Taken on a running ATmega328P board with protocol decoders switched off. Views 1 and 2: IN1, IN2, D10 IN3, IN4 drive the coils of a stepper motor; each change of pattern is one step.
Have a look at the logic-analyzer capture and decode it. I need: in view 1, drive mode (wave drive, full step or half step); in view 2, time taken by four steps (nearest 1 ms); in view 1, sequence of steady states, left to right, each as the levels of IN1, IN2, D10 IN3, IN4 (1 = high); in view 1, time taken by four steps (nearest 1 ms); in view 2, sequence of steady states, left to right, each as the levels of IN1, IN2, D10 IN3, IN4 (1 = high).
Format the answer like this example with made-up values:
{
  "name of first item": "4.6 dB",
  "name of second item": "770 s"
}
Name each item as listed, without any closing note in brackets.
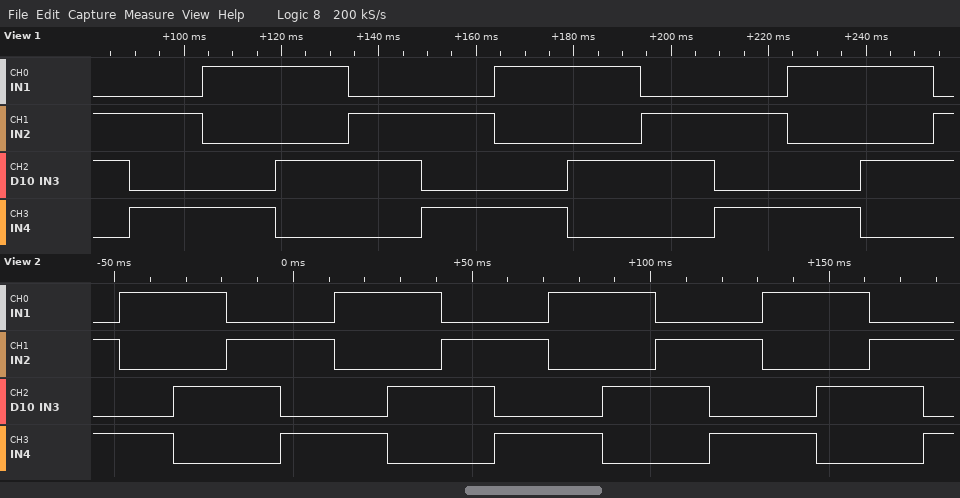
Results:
{
  "in view 1, drive mode": "full step",
  "in view 2, time taken by four steps": "60 ms",
  "in view 1, sequence of steady states, left to right, each as the levels of IN1, IN2, D10 IN3, IN4": "0110 0101 1001 1010 0110 0101 1001 1010 0110 0101 1001 1010 0110",
  "in view 1, time taken by four steps": "60 ms",
  "in view 2, sequence of steady states, left to right, each as the levels of IN1, IN2, D10 IN3, IN4": "0101 1001 1010 0110 0101 1001 1010 0110 0101 1001 1010 0110 0101 1001 1010 0110 0101"
}
